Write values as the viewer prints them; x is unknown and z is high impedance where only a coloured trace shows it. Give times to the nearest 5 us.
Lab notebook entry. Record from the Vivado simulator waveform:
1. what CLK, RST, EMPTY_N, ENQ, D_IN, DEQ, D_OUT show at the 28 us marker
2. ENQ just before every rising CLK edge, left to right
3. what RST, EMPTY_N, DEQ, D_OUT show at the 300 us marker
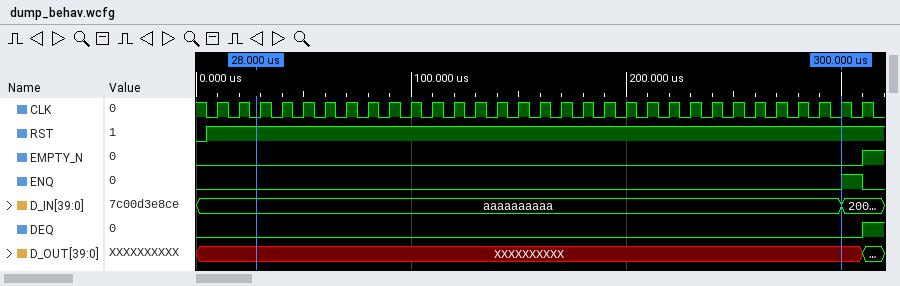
CLK=0, RST=1, EMPTY_N=0, ENQ=0, D_IN=aaaaaaaaaa, DEQ=0, D_OUT=XXXXXXXXXX
0 0 0 0 0 0 0 0 0 0 0 0 0 0 0 0 0 0 0 0 0 0 0 0 0 0 0 0 0 0 1
RST=1, EMPTY_N=0, DEQ=0, D_OUT=XXXXXXXXXX
